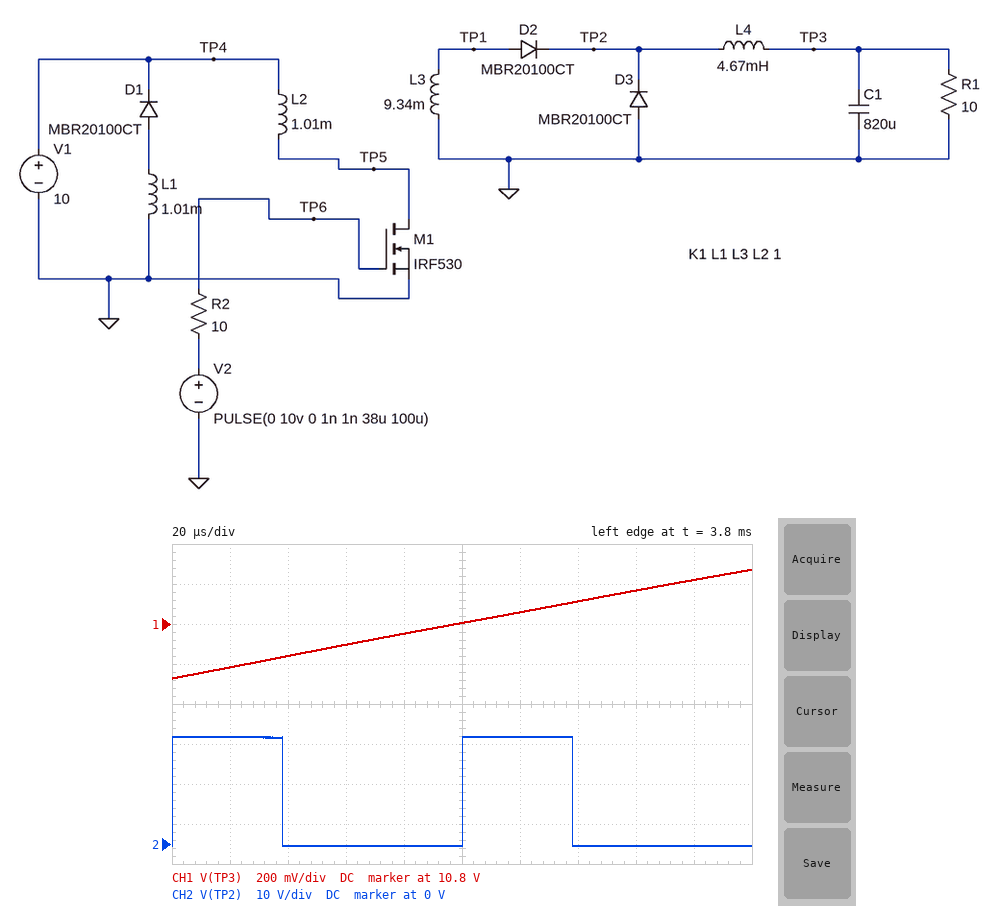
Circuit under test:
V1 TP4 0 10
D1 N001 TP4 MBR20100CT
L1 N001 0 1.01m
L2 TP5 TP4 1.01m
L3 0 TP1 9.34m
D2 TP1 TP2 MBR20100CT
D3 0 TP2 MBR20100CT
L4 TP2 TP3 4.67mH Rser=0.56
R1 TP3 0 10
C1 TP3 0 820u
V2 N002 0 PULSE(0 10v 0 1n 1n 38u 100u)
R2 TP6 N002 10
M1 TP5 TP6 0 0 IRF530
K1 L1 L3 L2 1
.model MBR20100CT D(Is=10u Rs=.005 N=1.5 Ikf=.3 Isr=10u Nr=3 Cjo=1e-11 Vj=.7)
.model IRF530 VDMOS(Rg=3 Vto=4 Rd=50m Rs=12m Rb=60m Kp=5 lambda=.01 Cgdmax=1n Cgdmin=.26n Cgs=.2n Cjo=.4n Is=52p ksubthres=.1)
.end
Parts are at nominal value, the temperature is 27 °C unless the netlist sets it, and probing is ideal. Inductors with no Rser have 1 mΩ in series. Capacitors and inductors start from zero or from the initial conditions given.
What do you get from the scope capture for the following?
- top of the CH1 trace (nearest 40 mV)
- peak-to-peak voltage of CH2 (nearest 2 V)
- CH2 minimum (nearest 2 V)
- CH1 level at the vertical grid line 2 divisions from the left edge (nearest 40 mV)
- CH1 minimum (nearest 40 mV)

11.08 V
28 V
0 V
10.64 V
10.52 V
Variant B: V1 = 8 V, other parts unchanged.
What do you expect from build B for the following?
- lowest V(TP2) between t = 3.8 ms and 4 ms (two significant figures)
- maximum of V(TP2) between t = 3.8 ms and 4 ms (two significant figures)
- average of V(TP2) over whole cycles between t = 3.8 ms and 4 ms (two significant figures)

-590 mV
21 V
7.7 V
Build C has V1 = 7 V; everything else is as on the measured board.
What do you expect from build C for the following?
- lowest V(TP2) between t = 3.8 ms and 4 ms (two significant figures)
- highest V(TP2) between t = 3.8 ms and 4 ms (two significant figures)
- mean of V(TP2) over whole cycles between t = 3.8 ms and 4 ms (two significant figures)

-580 mV
19 V
6.7 V
